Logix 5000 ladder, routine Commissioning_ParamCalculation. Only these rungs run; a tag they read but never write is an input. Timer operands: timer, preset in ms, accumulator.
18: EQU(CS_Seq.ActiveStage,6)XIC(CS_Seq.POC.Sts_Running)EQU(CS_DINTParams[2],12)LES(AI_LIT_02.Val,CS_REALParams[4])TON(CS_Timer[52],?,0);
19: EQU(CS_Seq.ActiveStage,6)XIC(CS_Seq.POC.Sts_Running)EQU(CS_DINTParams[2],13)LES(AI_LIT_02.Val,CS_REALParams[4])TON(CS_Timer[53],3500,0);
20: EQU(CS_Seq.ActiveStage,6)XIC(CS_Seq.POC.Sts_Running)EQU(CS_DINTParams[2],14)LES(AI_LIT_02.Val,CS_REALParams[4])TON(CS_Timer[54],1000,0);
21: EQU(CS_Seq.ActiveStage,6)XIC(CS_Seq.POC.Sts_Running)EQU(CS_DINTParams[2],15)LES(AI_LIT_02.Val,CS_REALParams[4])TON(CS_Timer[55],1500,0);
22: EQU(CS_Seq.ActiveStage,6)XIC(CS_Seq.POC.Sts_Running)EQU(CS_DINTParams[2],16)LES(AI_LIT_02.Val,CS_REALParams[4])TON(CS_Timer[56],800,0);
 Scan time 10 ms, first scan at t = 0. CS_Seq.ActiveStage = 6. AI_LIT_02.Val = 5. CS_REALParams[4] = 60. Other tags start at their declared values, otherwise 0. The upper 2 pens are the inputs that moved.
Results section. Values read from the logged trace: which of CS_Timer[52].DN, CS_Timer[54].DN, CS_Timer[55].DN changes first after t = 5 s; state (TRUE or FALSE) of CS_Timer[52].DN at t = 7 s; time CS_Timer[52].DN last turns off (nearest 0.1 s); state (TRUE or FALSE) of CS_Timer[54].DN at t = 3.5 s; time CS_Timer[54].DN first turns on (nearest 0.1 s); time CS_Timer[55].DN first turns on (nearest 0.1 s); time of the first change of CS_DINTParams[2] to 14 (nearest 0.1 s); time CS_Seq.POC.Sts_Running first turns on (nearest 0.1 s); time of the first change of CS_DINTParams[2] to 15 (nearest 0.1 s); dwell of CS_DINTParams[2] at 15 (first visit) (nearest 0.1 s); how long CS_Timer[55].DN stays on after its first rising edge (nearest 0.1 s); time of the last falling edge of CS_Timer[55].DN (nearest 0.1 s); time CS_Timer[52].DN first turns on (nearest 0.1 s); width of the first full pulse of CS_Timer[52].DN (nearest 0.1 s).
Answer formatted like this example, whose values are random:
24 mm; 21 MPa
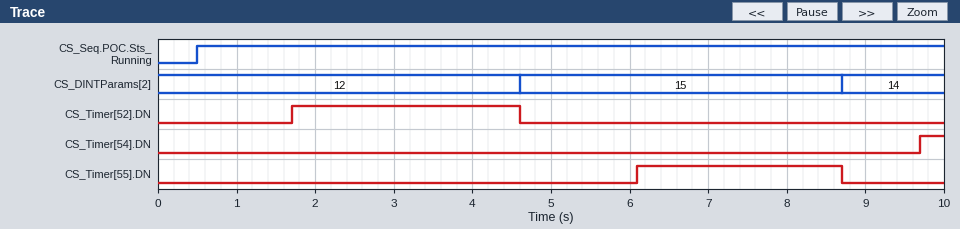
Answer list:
CS_Timer[55].DN; FALSE; 4.6 s; FALSE; 9.7 s; 6.1 s; 8.7 s; 0.5 s; 4.6 s; 4.1 s; 2.6 s; 8.7 s; 1.7 s; 2.9 s
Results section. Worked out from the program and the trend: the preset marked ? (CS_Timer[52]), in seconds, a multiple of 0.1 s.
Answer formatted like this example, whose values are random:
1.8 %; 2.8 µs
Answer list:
1.2 s
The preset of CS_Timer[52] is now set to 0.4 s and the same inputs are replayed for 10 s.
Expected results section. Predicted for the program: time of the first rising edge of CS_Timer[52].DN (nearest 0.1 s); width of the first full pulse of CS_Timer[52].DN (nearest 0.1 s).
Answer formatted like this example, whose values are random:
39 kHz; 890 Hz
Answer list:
0.9 s; 3.7 s
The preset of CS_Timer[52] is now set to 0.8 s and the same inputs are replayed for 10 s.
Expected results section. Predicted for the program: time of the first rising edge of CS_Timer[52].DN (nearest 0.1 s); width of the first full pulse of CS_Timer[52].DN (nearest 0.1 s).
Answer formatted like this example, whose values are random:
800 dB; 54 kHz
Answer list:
1.3 s; 3.3 s
